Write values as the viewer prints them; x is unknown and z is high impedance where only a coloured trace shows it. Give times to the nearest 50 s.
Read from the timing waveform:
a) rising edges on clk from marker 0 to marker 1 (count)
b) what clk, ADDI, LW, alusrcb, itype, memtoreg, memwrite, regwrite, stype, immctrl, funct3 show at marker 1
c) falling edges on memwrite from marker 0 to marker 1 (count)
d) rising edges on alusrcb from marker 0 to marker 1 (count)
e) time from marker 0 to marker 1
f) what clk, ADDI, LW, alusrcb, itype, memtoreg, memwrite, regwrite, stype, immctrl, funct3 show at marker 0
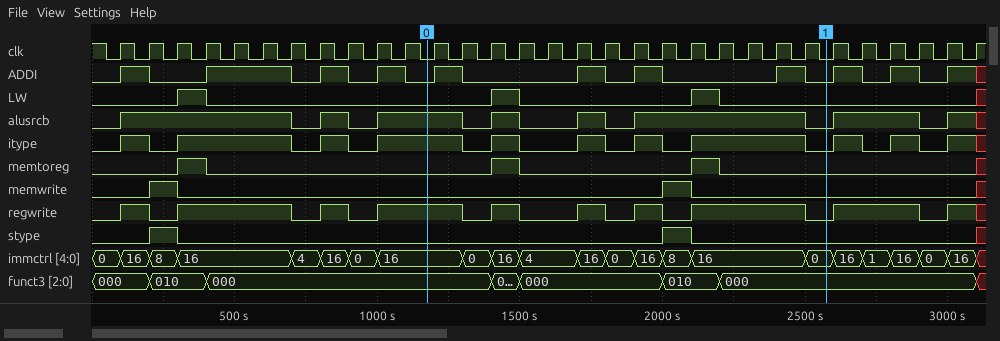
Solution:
14
clk=0, ADDI=0, LW=0, alusrcb=0, itype=0, memtoreg=0, memwrite=0, regwrite=0, stype=0, immctrl=0, funct3=000
1
3
1400 s
clk=0, ADDI=0, LW=0, alusrcb=1, itype=1, memtoreg=0, memwrite=0, regwrite=1, stype=0, immctrl=16, funct3=000
